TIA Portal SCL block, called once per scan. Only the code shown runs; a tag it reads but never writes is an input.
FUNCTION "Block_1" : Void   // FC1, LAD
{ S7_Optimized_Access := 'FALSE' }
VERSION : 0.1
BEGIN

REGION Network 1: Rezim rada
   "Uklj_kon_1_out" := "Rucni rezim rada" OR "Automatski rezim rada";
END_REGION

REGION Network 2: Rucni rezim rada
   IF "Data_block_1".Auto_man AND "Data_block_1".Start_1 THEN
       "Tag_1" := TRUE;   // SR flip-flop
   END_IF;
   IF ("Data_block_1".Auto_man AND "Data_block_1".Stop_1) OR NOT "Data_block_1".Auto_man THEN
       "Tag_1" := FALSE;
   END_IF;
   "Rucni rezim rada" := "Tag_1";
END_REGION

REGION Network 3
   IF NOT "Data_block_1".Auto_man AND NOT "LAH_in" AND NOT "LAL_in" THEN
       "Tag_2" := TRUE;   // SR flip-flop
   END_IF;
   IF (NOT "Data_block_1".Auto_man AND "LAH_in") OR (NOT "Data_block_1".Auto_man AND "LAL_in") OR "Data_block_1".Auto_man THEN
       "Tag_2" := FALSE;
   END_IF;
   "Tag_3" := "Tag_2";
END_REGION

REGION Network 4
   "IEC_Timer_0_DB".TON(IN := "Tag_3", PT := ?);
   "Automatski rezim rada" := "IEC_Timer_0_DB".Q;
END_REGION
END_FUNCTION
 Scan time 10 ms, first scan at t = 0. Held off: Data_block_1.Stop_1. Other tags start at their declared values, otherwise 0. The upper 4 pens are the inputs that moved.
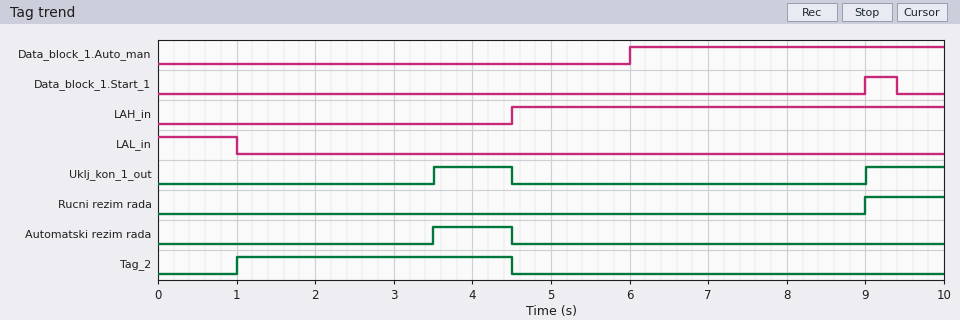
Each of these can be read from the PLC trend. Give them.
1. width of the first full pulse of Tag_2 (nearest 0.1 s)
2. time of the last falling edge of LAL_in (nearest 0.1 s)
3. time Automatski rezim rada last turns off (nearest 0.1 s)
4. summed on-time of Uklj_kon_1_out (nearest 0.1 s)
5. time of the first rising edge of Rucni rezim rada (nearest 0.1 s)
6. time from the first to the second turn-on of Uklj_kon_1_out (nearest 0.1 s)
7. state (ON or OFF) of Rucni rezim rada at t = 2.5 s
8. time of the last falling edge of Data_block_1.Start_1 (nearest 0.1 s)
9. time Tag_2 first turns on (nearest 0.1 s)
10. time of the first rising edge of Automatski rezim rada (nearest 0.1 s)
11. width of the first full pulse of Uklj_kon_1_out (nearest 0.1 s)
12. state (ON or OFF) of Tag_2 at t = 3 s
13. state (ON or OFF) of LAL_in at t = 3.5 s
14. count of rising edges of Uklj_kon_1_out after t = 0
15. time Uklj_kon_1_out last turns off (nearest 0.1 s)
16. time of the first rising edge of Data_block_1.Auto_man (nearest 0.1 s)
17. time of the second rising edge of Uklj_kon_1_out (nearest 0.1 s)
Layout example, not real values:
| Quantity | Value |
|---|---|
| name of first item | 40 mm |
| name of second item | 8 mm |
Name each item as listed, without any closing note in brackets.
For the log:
| Quantity | Value |
|---|---|
| width of the first full pulse of Tag_2 | 3.5 s |
| time of the last falling edge of LAL_in | 1.0 s |
| time Automatski rezim rada last turns off | 4.5 s |
| summed on-time of Uklj_kon_1_out | 2.0 s |
| time of the first rising edge of Rucni rezim rada | 9.0 s |
| time from the first to the second turn-on of Uklj_kon_1_out | 5.5 s |
| state (ON or OFF) of Rucni rezim rada at t = 2.5 s | OFF |
| time of the last falling edge of Data_block_1.Start_1 | 9.4 s |
| time Tag_2 first turns on | 1.0 s |
| time of the first rising edge of Automatski rezim rada | 3.5 s |
| width of the first full pulse of Uklj_kon_1_out | 1.0 s |
| state (ON or OFF) of Tag_2 at t = 3 s | ON |
| state (ON or OFF) of LAL_in at t = 3.5 s | OFF |
| count of rising edges of Uklj_kon_1_out after t = 0 | 2 |
| time Uklj_kon_1_out last turns off | 4.5 s |
| time of the first rising edge of Data_block_1.Auto_man | 6.0 s |
| time of the second rising edge of Uklj_kon_1_out | 9.0 s |
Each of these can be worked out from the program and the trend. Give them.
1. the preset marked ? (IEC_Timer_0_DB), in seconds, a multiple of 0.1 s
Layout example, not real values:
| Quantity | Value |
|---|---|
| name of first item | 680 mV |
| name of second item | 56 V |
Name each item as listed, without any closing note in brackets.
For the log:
| Quantity | Value |
|---|---|
| the preset marked ? (IEC_Timer_0_DB), in seconds, a multiple of 0.1 s | 2.5 s |
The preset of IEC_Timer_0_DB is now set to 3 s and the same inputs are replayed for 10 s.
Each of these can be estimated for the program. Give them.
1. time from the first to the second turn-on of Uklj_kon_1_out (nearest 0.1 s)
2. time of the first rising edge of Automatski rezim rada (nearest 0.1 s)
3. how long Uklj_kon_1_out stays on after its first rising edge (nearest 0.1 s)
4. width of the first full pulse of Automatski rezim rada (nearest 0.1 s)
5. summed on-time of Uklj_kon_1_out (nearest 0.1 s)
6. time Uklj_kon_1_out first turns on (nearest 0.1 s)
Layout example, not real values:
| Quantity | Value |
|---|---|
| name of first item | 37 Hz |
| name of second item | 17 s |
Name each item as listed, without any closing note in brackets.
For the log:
| Quantity | Value |
|---|---|
| time from the first to the second turn-on of Uklj_kon_1_out | 5.0 s |
| time of the first rising edge of Automatski rezim rada | 4.0 s |
| how long Uklj_kon_1_out stays on after its first rising edge | 0.5 s |
| width of the first full pulse of Automatski rezim rada | 0.5 s |
| summed on-time of Uklj_kon_1_out | 1.5 s |
| time Uklj_kon_1_out first turns on | 4.0 s |
